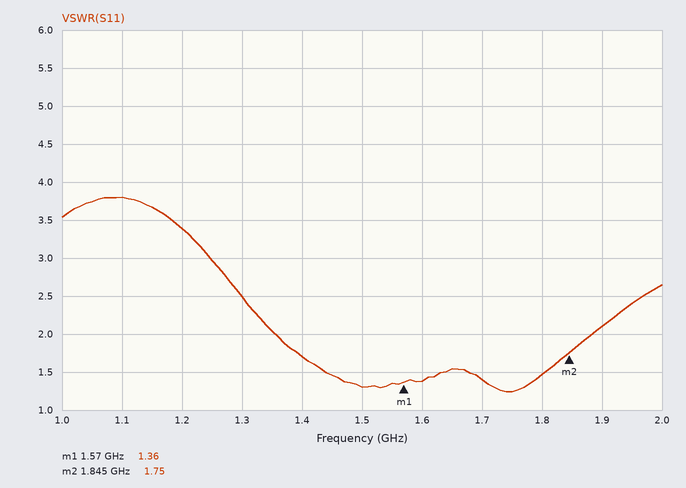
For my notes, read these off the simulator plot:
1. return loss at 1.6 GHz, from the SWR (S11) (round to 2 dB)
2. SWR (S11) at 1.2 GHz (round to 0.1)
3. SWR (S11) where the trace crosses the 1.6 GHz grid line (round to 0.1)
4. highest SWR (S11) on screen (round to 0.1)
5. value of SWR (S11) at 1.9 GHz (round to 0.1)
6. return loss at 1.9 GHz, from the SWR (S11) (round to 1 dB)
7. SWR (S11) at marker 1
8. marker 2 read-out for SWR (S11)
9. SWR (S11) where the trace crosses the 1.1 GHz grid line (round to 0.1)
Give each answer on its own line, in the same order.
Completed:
16 dB
3.4
1.4
3.8
2.1
9 dB
1.36
1.75
3.8
